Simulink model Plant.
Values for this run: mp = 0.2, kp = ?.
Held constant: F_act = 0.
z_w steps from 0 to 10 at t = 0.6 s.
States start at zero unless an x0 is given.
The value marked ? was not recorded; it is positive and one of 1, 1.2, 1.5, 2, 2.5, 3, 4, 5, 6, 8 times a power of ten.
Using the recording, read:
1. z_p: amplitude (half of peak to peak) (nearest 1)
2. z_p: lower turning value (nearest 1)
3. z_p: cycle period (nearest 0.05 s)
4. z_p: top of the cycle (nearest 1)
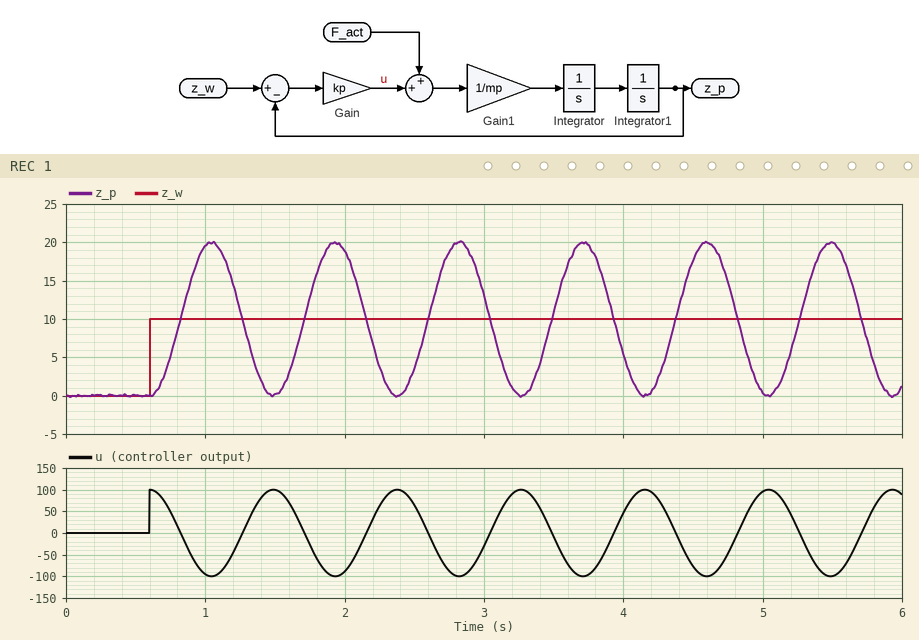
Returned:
10
0
0.90 s
20
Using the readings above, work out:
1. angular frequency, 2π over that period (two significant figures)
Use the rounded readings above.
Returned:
7.0 rad/s
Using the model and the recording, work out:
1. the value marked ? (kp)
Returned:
10
